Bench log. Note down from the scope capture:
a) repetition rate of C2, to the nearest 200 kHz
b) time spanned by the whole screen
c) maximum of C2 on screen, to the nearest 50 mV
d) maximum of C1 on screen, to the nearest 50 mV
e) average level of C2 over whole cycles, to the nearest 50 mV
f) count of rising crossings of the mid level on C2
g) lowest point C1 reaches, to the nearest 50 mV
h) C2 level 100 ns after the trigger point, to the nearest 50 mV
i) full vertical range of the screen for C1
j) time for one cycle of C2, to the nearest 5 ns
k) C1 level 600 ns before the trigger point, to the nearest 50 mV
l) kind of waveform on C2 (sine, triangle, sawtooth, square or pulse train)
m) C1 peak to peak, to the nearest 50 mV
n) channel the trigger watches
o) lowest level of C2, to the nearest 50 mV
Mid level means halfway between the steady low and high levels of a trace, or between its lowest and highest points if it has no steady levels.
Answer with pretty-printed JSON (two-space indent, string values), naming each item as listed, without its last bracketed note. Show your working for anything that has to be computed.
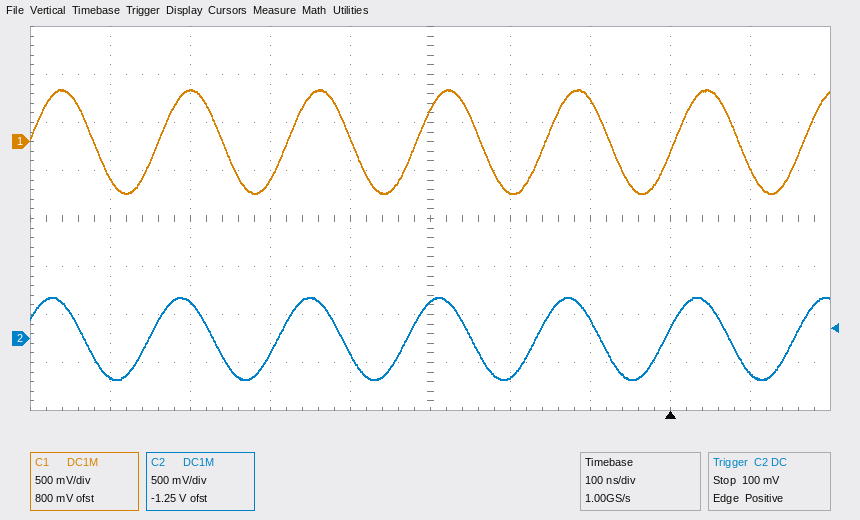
{
  "repetition rate of C2, to the nearest 200 kHz": "1 / 160 ns ≈ 6.2 MHz",
  "time spanned by the whole screen": "1 µs",
  "maximum of C2 on screen, to the nearest 50 mV": "450 mV",
  "maximum of C1 on screen, to the nearest 50 mV": "550 mV",
  "average level of C2 over whole cycles, to the nearest 50 mV": "(450 mV + (-450 mV)) / 2 ≈ 0 mV",
  "count of rising crossings of the mid level on C2": "6",
  "lowest point C1 reaches, to the nearest 50 mV": "-550 mV",
  "C2 level 100 ns after the trigger point, to the nearest 50 mV": "-350 mV",
  "full vertical range of the screen for C1": "4 V",
  "time for one cycle of C2, to the nearest 5 ns": "160 ns",
  "C1 level 600 ns before the trigger point, to the nearest 50 mV": "550 mV",
  "kind of waveform on C2": "sine",
  "C1 peak to peak, to the nearest 50 mV": "550 mV − (-550 mV) = 1.10 V",
  "channel the trigger watches": "C2",
  "lowest level of C2, to the nearest 50 mV": "-450 mV"
}
